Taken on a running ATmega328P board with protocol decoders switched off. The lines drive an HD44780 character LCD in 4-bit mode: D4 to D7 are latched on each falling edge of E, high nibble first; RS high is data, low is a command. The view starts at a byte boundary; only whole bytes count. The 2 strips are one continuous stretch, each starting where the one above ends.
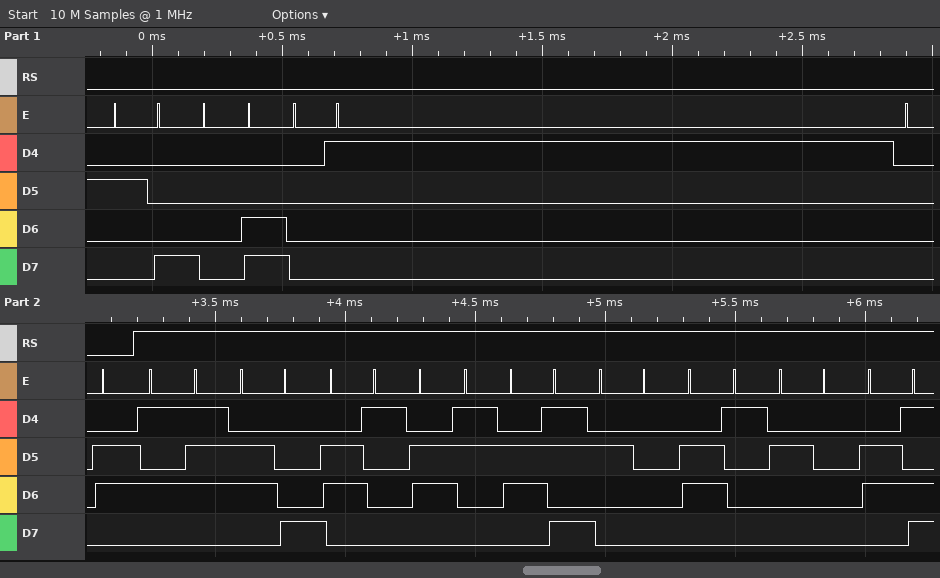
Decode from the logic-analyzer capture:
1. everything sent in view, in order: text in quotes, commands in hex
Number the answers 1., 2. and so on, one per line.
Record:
1. 0x28 0x0C 0x01 0x06 "Whack a m"
